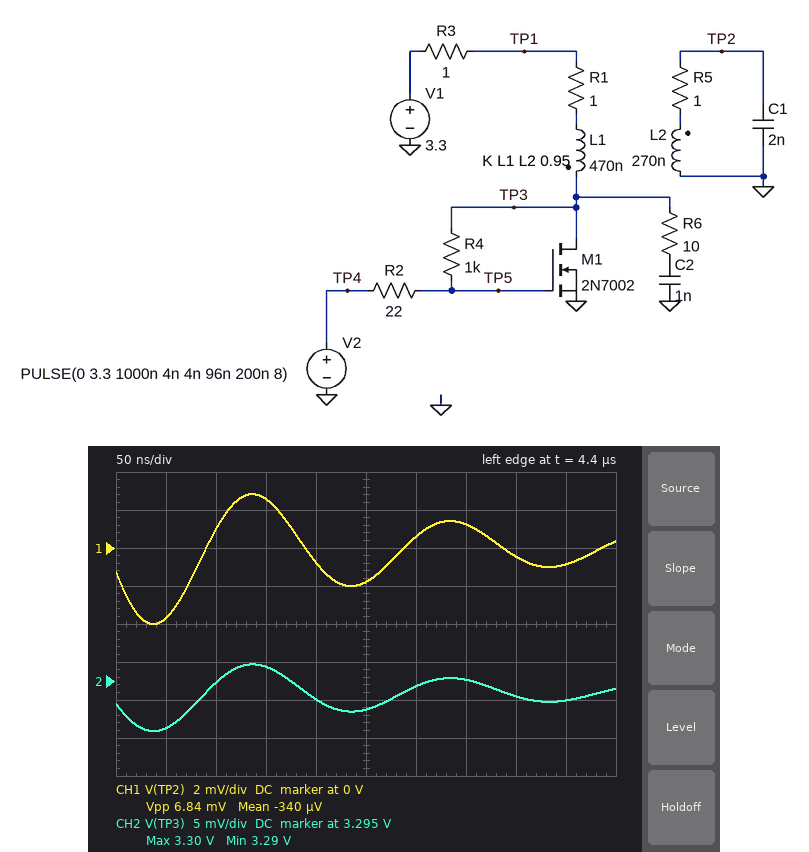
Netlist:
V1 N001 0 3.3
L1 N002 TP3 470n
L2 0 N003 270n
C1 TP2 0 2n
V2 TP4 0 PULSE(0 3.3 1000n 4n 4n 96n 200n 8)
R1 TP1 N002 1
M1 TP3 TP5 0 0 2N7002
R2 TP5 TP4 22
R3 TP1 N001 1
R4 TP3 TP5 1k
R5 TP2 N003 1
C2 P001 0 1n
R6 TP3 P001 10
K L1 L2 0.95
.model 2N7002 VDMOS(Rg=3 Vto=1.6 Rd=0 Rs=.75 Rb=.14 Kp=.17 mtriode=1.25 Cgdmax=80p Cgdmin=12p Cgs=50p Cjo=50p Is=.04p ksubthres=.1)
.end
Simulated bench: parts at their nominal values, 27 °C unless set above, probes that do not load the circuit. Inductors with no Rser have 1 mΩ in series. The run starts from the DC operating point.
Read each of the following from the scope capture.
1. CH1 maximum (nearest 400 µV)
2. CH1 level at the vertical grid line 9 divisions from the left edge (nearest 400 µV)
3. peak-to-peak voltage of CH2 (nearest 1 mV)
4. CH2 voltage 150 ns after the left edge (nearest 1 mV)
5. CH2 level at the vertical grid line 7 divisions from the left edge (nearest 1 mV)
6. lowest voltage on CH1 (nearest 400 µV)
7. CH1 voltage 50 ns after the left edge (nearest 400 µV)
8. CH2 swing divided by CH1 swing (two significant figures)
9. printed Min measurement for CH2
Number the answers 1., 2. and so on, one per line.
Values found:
1. 2.8 mV
2. -800 µV
3. 9 mV
4. 3.297 V
5. 3.295 V
6. -4.0 mV
7. -3.6 mV
8. 1.3
9. 3.29 V
